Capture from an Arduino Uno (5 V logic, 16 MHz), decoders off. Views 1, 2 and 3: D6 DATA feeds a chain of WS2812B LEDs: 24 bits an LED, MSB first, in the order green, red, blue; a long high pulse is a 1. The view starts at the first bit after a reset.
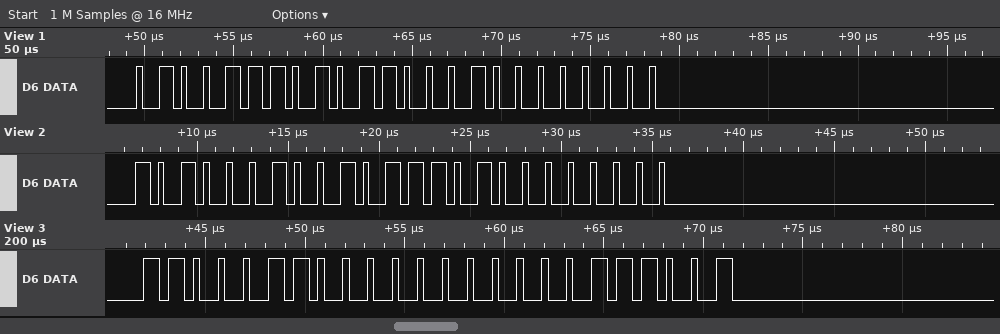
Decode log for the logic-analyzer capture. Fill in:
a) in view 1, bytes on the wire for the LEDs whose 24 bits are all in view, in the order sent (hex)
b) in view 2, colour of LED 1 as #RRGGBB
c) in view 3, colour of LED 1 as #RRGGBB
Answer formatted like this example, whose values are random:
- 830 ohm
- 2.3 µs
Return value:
- 4E B1 00
- #5DA200
- #00C639
